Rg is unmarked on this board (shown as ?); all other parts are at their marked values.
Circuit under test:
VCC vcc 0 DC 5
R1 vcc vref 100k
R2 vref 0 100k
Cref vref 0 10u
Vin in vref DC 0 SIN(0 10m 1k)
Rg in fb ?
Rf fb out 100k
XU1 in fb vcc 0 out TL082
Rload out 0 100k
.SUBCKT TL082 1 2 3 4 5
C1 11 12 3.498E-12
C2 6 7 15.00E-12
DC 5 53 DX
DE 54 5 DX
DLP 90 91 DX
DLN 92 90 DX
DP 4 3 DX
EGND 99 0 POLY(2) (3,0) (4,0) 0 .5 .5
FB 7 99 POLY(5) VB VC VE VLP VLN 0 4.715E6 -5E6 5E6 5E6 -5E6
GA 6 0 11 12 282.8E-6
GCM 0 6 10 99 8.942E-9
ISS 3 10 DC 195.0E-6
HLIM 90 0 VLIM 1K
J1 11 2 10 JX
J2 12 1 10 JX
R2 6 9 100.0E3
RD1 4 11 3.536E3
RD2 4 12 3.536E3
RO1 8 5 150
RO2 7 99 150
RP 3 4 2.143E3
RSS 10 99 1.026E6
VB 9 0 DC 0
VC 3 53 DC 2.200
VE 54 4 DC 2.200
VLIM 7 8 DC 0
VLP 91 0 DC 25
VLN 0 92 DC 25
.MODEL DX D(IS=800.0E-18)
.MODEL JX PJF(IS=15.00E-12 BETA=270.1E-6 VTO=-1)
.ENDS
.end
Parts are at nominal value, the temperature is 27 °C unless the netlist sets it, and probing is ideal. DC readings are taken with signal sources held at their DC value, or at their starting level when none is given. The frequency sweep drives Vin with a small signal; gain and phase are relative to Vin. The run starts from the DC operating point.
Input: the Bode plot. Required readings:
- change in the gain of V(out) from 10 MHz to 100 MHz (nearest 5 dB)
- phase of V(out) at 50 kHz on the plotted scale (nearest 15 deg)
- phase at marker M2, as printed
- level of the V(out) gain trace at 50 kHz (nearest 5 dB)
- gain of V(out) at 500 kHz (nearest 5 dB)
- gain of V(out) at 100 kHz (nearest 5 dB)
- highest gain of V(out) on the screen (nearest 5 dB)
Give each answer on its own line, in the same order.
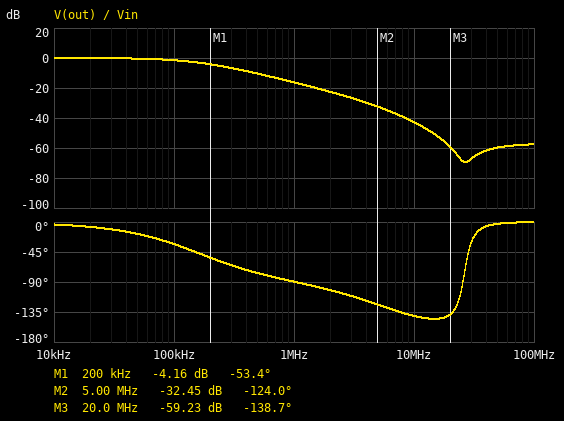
-15 dB
-15 deg
-124.0 deg
0 dB
-10 dB
0 dB
0 dB
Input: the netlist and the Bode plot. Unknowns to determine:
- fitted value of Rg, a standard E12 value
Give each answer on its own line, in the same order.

4.7 kΩ
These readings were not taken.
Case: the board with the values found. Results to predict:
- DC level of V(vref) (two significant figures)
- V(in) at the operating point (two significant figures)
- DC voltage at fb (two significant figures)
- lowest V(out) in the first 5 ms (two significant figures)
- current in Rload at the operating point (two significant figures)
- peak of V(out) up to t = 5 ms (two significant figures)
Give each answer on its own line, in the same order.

2.5 V
2.5 V
2.5 V
2.5 V
25 µA
2.5 V
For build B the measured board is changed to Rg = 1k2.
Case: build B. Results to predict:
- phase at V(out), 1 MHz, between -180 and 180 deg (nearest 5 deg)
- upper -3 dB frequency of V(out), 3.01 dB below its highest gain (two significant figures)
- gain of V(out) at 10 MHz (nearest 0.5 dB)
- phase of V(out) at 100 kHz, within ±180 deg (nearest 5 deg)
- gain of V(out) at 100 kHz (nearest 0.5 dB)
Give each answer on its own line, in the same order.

-95 deg
41 kHz
-58.0 dB
-70 deg
-8.5 dB
